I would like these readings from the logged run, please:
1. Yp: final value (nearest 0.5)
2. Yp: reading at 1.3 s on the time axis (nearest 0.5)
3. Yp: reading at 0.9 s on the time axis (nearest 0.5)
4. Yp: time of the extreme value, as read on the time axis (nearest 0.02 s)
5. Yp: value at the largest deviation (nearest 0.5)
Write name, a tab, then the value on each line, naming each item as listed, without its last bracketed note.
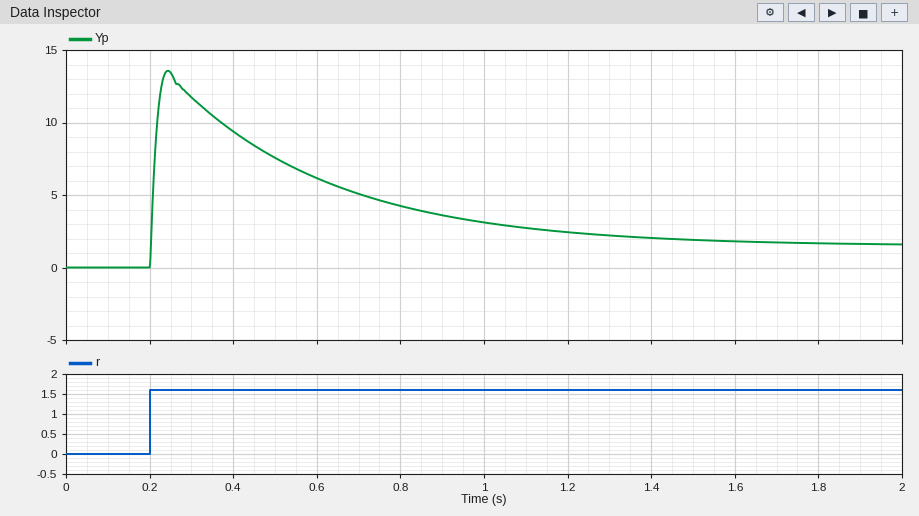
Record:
Yp: final value	1.5
Yp: reading at 1.3 s on the time axis	2.0
Yp: reading at 0.9 s on the time axis	3.5
Yp: time of the extreme value, as read on the time axis	0.24 s
Yp: value at the largest deviation	13.5
